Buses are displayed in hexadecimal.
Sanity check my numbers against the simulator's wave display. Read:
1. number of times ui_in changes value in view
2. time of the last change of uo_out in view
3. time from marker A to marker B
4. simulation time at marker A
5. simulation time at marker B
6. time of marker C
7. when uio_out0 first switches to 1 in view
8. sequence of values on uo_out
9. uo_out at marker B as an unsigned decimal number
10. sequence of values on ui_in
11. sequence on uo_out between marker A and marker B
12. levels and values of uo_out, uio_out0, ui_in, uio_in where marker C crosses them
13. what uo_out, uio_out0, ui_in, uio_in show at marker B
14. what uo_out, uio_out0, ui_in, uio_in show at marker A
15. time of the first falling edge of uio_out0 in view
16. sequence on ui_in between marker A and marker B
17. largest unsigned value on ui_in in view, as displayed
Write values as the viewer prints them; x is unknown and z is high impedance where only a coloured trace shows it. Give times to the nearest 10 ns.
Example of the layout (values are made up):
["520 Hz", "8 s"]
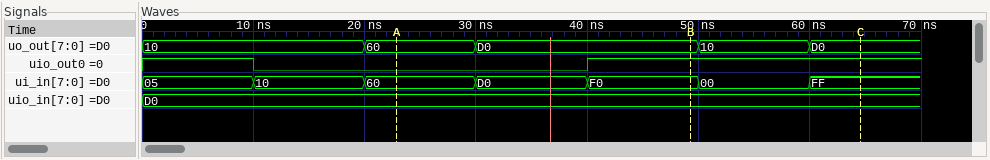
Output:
["6", "60 ns", "30 ns", "20 ns", "50 ns", "60 ns", "40 ns", "10, 60, D0, 10, D0", "208", "05, 10, 60, D0, F0, 00, FF", "60, D0", "uo_out=D0, uio_out0=1, ui_in=FF, uio_in=D0", "uo_out=D0, uio_out0=1, ui_in=F0, uio_in=D0", "uo_out=60, uio_out0=0, ui_in=60, uio_in=D0", "10 ns", "60, D0, F0", "FF"]
